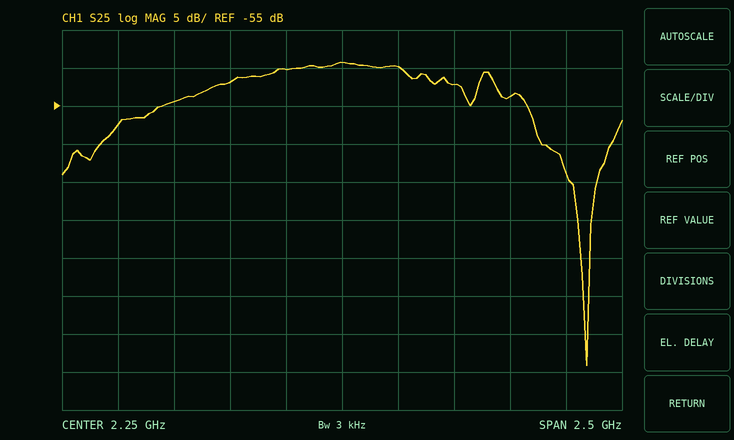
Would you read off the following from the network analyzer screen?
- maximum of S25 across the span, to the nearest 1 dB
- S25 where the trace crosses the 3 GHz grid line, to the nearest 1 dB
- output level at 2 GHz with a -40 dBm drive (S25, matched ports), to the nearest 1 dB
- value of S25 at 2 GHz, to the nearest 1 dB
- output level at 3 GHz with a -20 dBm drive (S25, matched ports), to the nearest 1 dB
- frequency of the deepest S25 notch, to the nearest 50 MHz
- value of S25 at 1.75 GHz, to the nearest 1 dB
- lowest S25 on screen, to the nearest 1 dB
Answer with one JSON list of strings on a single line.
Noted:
["-49 dB", "-54 dB", "-90 dBm", "-50 dB", "-74 dBm", "3.35 GHz", "-52 dB", "-89 dB"]
